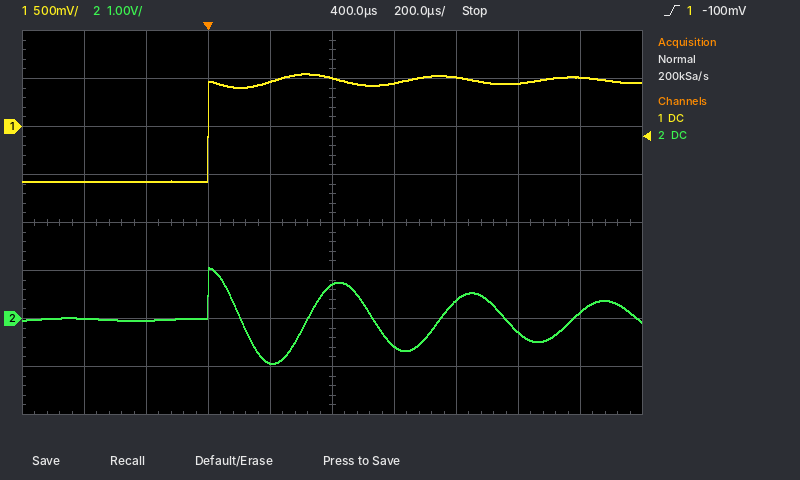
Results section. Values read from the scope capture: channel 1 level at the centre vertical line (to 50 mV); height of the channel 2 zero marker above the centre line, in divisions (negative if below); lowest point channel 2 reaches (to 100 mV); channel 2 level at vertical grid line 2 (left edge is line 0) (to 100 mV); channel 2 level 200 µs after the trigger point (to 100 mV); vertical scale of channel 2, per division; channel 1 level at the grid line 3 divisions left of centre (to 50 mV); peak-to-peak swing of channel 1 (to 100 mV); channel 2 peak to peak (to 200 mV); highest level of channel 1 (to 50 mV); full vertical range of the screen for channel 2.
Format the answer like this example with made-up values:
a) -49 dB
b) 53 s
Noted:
a) 500 mV
b) -2.0 div
c) -900 mV
d) 0.0 V
e) -900 mV
f) 1 V
g) -550 mV
h) 1.10 V
i) 2.0 V
j) 550 mV
k) 8 V
